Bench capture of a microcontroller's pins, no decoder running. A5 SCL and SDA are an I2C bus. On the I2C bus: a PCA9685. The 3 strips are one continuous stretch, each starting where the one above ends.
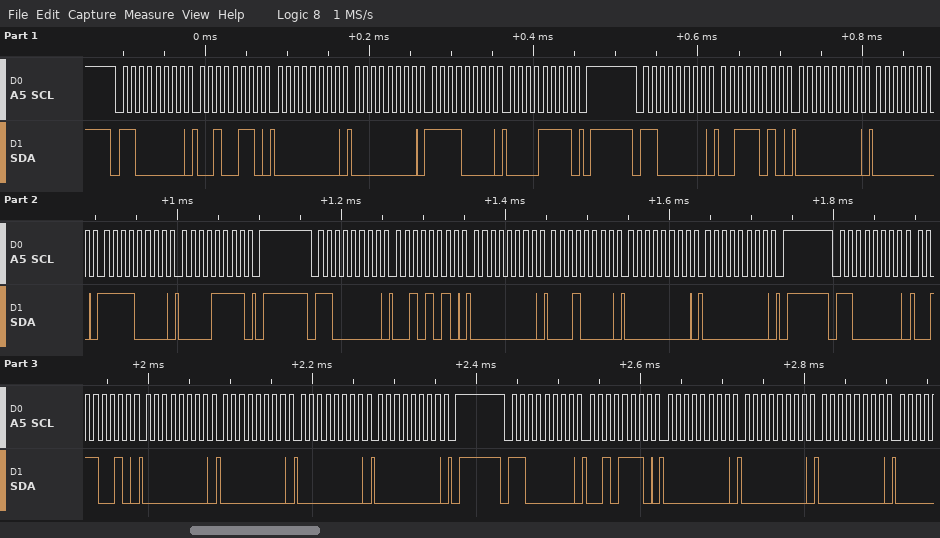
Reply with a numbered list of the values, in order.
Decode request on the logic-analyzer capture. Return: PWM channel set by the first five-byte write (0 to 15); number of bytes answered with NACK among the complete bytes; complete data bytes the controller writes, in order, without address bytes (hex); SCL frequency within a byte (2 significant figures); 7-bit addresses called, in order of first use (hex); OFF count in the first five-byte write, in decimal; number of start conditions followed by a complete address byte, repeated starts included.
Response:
1. 8
2. 0
3. 26 00 00 F0 0F 3A 00 00 F0 0F 2A 00 10 00 00 32 00 00 00 00 2E 00 00 00
4. 100 kHz
5. 0x60
6. 4080
7. 5
